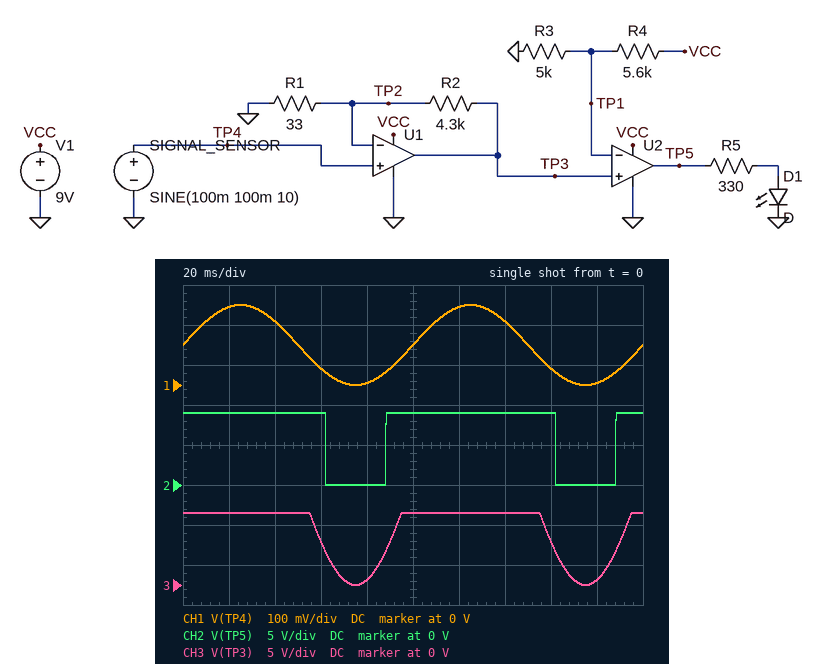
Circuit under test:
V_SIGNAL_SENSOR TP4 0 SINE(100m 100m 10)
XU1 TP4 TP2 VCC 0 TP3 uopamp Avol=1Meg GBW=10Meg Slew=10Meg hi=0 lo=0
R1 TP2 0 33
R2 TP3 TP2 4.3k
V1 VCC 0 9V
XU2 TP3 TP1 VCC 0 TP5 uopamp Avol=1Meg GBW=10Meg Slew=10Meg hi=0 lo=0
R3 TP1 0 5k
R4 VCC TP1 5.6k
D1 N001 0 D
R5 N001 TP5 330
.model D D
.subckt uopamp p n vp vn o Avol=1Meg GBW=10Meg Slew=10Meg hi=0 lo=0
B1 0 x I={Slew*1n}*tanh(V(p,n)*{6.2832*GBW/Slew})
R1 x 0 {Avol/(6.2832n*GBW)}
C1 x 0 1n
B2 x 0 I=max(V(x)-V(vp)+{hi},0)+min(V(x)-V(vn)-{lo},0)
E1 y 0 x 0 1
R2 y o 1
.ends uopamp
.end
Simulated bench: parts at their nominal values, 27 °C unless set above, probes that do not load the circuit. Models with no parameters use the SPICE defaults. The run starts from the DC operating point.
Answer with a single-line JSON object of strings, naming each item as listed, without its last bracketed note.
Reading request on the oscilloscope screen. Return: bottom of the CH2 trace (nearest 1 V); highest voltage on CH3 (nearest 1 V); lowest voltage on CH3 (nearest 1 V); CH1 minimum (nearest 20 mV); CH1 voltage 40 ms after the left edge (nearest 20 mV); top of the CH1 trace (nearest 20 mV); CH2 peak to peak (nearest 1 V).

{"bottom of the CH2 trace": "0 V", "highest voltage on CH3": "9 V", "lowest voltage on CH3": "0 V", "CH1 minimum": "0 V", "CH1 voltage 40 ms after the left edge": "160 mV", "top of the CH1 trace": "200 mV", "CH2 peak to peak": "9 V"}
